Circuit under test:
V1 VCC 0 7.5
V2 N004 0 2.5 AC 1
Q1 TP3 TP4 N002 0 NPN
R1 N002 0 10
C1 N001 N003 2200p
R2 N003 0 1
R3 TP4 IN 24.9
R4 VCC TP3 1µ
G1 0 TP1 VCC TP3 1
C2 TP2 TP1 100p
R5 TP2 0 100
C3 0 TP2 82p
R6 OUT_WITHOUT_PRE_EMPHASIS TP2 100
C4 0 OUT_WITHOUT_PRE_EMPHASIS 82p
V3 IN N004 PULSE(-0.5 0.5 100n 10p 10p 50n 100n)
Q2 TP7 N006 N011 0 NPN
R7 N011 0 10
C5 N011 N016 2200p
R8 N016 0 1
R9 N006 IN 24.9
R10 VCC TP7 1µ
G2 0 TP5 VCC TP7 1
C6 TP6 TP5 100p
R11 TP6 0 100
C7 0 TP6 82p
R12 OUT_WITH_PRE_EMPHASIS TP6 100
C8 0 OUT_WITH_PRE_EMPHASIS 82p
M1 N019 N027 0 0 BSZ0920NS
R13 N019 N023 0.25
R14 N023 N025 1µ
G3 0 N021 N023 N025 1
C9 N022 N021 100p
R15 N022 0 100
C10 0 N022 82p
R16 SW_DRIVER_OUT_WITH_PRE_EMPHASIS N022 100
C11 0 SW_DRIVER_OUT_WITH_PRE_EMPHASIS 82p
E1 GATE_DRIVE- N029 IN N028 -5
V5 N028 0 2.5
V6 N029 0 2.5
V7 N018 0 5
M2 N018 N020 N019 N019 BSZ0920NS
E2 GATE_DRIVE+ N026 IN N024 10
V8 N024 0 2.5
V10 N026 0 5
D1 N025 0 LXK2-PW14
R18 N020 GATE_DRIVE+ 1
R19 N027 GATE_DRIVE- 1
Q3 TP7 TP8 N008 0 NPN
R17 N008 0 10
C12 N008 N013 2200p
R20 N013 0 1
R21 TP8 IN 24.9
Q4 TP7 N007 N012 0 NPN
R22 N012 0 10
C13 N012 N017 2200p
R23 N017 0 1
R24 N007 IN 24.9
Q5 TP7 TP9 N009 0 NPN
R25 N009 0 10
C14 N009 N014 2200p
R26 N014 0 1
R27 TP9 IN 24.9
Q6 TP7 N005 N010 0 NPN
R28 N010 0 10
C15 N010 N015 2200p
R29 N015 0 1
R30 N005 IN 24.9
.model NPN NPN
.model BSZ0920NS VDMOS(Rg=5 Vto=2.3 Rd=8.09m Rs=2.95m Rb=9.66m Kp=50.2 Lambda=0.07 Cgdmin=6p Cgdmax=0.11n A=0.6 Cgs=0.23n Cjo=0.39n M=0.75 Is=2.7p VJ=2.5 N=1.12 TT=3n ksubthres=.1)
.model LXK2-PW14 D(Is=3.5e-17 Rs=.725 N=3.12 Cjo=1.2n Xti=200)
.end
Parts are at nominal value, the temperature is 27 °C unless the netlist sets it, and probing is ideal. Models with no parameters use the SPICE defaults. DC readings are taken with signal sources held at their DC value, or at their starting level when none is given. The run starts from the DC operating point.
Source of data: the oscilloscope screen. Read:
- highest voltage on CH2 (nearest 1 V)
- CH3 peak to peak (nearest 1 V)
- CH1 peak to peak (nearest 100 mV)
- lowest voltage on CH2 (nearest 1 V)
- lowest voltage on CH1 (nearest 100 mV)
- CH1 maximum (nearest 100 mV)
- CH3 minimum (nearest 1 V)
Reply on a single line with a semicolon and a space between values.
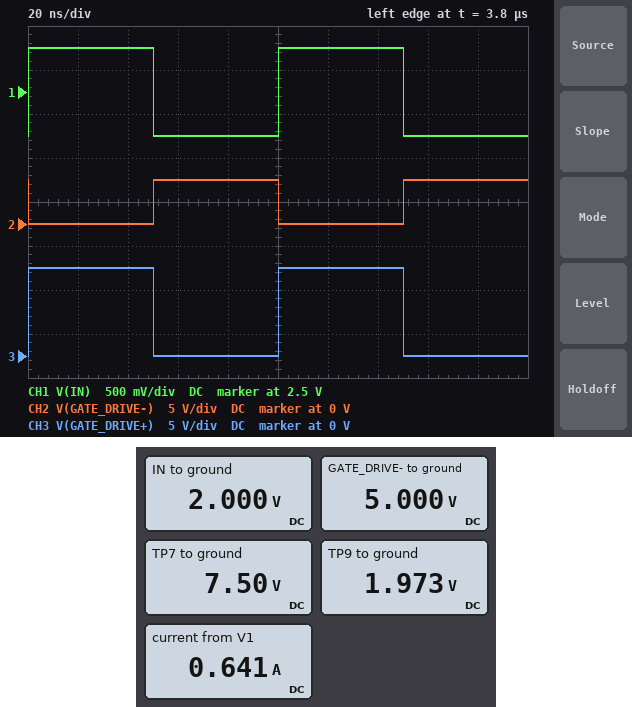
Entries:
5 V; 10 V; 1.0 V; 0 V; 2.0 V; 3.0 V; 0 V
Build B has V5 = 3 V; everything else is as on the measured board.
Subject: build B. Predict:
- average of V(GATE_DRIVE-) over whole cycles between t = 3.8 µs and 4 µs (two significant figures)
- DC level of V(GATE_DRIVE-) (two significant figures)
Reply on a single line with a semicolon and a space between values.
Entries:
5.0 V; 7.5 V
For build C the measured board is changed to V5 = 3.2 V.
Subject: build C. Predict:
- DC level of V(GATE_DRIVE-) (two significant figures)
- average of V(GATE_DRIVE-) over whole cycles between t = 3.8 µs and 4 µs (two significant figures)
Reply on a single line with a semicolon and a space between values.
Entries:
8.5 V; 6.0 V
